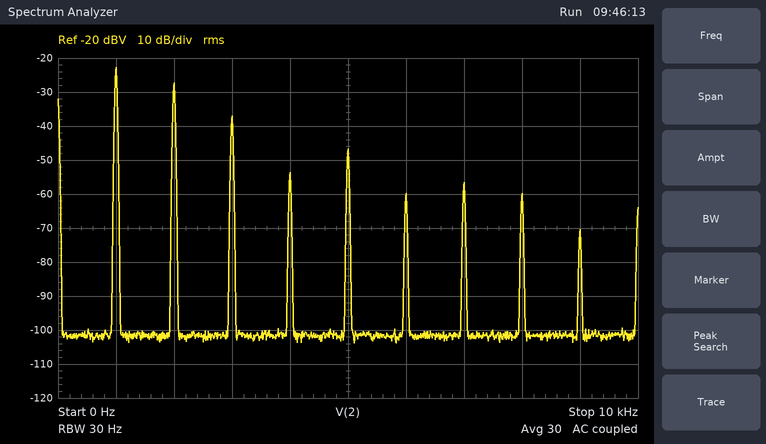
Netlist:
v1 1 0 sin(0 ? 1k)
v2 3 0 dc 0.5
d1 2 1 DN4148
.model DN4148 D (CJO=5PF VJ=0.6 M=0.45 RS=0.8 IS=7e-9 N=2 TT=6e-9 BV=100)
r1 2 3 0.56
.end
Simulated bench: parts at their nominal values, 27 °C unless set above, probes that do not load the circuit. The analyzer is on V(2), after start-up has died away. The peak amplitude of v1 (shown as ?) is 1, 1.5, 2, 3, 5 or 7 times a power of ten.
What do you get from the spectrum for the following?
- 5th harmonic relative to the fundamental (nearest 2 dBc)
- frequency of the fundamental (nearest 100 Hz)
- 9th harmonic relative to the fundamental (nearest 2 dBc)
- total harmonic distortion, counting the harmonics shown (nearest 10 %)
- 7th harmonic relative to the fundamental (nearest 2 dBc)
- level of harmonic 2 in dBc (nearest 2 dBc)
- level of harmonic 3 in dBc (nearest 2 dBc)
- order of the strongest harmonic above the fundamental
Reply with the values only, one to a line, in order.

-24 dBc
1.0 kHz
-48 dBc
60 %
-34 dBc
-4 dBc
-14 dBc
2
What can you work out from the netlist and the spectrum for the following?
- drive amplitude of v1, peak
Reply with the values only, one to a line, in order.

1 V
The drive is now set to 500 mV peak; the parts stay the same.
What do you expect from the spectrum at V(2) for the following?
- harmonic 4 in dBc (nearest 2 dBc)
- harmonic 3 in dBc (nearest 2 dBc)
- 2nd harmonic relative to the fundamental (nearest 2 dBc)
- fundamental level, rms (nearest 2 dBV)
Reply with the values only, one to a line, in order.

-20 dBc
-10 dBc
-4 dBc
-36 dBV
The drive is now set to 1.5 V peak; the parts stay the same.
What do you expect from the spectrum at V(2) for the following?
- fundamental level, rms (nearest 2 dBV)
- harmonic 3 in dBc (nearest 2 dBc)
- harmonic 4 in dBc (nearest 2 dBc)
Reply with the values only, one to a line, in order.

-18 dBV
-18 dBc
-24 dBc
